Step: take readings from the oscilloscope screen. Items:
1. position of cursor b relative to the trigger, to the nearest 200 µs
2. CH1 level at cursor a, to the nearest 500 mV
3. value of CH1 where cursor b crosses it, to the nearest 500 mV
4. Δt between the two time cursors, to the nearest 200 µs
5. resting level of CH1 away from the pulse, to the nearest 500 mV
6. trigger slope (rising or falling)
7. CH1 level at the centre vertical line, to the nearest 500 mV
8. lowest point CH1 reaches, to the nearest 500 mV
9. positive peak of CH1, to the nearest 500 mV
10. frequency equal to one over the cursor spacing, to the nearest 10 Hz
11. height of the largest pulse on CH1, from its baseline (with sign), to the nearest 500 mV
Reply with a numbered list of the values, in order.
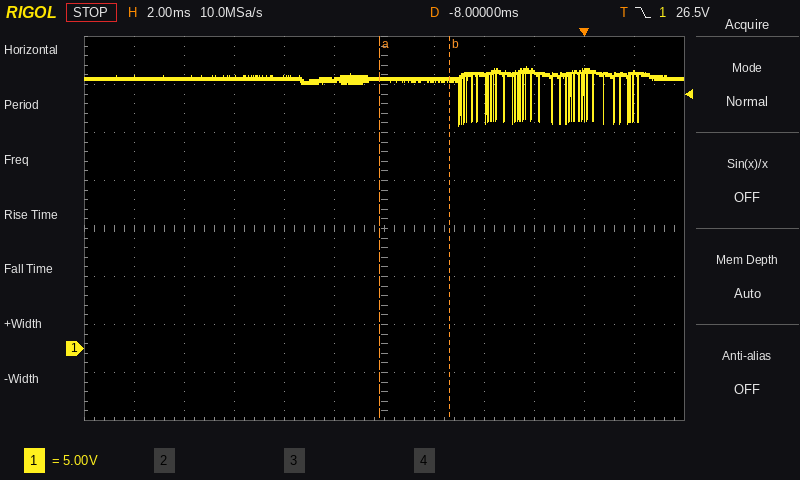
1. -5.4 ms
2. 28.0 V
3. 28.0 V
4. 2.8 ms
5. 28.0 V
6. falling
7. 28.0 V
8. 23.0 V
9. 29.5 V
10. 360 Hz
11. -5.0 V
